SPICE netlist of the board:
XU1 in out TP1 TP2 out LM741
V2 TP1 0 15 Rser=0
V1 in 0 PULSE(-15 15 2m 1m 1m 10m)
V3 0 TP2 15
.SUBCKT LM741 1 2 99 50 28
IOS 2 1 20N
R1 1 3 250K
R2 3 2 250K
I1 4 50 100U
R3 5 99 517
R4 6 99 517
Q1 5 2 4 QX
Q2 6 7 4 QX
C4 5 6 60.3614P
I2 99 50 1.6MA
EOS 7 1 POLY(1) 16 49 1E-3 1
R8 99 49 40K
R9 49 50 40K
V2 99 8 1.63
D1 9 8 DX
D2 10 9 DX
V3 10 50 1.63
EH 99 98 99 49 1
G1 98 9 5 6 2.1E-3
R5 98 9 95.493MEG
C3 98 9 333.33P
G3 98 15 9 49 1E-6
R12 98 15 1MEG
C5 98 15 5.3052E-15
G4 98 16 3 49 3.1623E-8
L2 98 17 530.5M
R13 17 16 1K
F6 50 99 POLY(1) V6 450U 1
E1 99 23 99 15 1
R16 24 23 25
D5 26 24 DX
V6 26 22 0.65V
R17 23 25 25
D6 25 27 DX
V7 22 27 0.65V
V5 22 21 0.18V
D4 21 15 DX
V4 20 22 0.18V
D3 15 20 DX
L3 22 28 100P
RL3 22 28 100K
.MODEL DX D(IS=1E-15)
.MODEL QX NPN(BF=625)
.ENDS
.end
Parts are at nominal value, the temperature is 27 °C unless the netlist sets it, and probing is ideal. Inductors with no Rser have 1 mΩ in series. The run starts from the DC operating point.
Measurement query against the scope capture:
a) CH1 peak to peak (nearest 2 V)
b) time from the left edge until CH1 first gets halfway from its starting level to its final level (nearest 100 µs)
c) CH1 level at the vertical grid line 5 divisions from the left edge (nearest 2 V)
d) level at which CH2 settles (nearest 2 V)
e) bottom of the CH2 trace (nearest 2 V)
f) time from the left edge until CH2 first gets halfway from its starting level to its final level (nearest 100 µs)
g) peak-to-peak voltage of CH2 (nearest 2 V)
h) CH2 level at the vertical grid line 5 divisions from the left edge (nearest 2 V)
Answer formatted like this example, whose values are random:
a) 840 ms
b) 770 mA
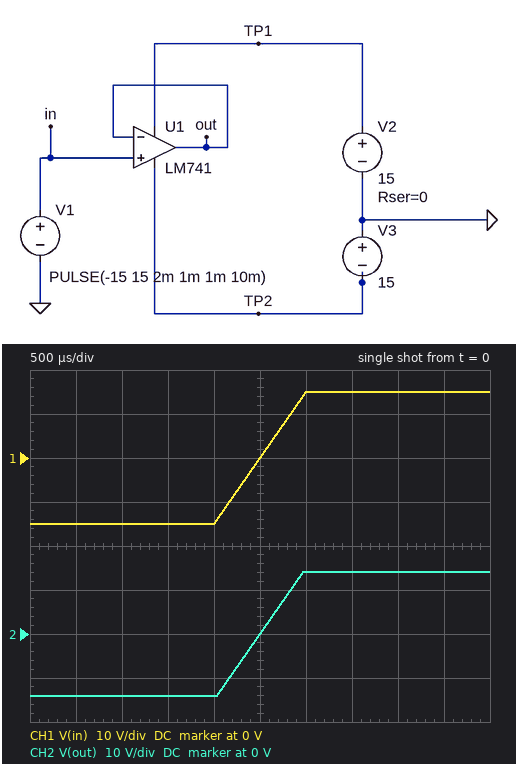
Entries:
a) 30 V
b) 2.5 ms
c) 0 V
d) 14 V
e) -14 V
f) 2.5 ms
g) 28 V
h) 0 V
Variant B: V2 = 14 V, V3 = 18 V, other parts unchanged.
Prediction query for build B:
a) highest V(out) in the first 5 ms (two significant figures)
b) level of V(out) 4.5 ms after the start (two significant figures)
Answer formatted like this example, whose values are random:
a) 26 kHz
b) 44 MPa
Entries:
a) 13 V
b) -17 V
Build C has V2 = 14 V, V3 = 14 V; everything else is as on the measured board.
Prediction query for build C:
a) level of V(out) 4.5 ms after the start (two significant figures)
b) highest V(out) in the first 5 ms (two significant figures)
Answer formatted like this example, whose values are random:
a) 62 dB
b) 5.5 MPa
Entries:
a) -13 V
b) 13 V
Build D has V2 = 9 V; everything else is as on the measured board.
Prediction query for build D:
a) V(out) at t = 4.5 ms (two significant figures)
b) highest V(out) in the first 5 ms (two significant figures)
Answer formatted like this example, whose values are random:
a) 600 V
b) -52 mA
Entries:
a) -14 V
b) 8.0 V
